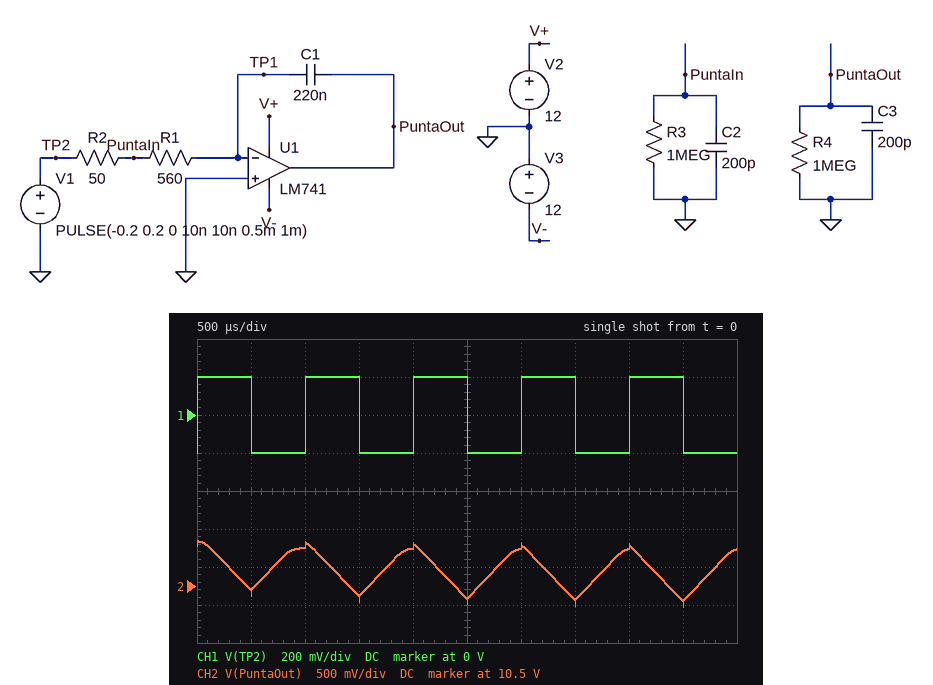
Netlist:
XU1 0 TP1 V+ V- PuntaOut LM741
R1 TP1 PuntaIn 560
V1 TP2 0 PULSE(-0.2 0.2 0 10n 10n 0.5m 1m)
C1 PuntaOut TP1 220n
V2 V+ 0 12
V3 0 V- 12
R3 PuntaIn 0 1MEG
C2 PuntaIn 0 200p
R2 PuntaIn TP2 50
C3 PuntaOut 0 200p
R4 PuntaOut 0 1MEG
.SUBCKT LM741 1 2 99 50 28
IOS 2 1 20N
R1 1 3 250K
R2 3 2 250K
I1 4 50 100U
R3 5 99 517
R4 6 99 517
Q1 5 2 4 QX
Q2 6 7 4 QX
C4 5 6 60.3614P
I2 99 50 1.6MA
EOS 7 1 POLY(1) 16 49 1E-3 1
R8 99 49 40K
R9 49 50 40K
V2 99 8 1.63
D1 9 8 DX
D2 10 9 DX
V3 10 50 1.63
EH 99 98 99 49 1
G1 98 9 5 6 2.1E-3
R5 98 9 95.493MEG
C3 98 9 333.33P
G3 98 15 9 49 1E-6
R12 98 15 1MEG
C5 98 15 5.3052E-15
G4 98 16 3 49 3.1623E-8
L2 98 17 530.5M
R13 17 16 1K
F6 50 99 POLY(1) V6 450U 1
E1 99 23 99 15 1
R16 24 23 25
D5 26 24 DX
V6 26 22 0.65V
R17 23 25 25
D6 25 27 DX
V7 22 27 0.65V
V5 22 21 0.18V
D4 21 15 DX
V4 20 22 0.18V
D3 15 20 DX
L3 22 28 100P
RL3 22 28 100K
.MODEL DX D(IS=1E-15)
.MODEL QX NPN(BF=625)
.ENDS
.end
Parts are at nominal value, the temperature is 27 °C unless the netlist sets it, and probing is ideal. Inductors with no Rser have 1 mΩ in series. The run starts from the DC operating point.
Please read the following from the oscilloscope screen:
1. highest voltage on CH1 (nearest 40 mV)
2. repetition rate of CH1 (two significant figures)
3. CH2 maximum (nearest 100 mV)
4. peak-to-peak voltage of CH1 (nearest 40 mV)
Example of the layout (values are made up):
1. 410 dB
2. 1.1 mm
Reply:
1. 200 mV
2. 1.0 kHz
3. 11.1 V
4. 400 mV
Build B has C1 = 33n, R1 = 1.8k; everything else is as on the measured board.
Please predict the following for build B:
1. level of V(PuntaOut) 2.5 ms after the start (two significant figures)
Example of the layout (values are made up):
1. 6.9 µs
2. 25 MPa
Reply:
1. 9.5 V
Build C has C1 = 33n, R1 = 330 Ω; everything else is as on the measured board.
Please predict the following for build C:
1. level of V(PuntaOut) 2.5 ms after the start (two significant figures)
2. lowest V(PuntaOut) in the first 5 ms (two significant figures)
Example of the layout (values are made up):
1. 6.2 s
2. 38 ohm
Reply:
1. 3.3 V
2. 3.2 V
